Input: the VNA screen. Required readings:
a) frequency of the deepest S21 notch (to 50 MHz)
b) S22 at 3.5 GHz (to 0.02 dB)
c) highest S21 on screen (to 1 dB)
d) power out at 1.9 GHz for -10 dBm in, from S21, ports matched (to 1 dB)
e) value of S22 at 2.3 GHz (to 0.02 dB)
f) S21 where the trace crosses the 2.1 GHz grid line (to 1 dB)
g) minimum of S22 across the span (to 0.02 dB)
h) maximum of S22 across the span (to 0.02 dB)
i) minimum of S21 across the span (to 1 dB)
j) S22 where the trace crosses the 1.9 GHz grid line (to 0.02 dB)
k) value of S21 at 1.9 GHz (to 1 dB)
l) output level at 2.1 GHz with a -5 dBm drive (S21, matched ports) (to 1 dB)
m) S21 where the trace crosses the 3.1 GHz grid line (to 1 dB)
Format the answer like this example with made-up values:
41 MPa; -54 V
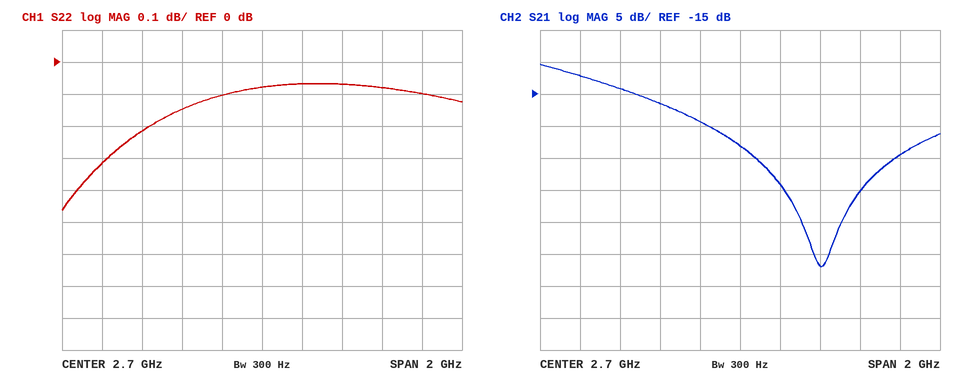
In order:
3.10 GHz; -0.10 dB; -10 dB; -22 dBm; -0.14 dB; -14 dB; -0.46 dB; -0.06 dB; -42 dB; -0.32 dB; -12 dB; -19 dBm; -42 dB
